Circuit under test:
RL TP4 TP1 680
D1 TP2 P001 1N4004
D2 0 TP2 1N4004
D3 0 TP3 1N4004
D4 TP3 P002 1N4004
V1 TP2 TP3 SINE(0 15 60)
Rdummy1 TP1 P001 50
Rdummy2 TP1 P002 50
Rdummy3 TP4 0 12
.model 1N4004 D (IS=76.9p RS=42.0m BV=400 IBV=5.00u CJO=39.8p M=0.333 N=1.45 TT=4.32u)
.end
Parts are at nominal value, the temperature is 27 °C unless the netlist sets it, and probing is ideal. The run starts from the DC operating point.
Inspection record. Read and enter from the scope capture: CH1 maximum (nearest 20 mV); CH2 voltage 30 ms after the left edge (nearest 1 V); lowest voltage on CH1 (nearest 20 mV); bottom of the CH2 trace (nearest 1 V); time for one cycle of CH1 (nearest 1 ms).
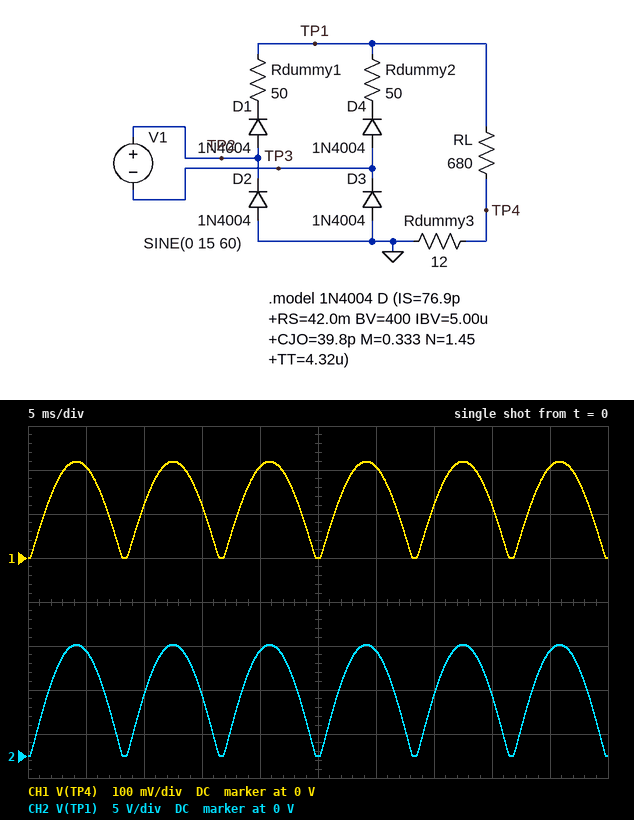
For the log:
220 mV
12 V
0 V
0 V
8 ms
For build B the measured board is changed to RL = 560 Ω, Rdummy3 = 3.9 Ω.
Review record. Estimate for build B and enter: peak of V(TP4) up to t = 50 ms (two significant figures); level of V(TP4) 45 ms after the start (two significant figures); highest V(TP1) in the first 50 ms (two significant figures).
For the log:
86 mV
81 mV
12 V
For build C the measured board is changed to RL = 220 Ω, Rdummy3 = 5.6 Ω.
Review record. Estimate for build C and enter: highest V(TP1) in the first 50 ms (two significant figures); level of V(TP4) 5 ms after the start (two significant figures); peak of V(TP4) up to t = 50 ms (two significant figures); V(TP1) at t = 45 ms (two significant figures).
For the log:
11 V
260 mV
270 mV
10 V
